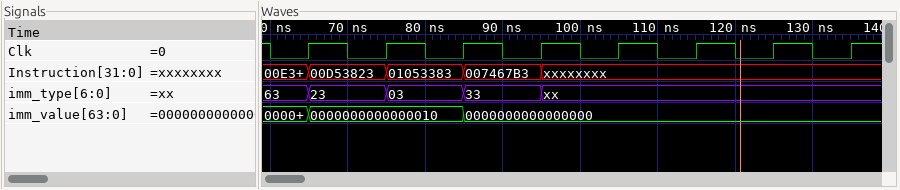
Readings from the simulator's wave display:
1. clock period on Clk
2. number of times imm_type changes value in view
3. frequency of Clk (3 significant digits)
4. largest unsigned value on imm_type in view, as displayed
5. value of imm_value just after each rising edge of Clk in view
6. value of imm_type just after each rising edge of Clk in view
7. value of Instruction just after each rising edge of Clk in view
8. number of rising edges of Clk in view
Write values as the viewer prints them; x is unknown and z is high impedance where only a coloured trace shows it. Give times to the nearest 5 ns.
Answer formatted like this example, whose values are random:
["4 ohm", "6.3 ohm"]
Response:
["10 ns", "4", "100 MHz", "63", "0000000000000010, 0000000000000010, 0000000000000000, 0000000000000000, 0000000000000000, 0000000000000000, 0000000000000000, 0000000000000000", "23, 03, 33, xx, xx, xx, xx, xx", "00D53823, 01053383, 007467B3, xxxxxxxx, xxxxxxxx, xxxxxxxx, xxxxxxxx, xxxxxxxx", "8"]
